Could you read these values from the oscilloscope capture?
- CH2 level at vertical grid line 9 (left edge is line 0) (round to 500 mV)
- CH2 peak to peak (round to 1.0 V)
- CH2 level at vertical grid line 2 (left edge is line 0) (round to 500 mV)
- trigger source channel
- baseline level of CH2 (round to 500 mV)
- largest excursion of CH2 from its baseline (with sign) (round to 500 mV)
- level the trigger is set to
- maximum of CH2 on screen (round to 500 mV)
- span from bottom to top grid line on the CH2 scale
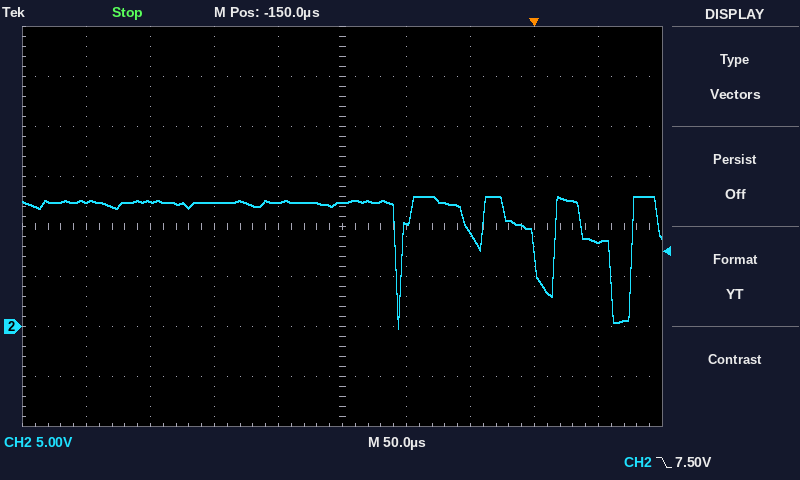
8.5 V
13.0 V
12.5 V
CH2
12.5 V
-12.5 V
7.50 V
13.0 V
40 V
